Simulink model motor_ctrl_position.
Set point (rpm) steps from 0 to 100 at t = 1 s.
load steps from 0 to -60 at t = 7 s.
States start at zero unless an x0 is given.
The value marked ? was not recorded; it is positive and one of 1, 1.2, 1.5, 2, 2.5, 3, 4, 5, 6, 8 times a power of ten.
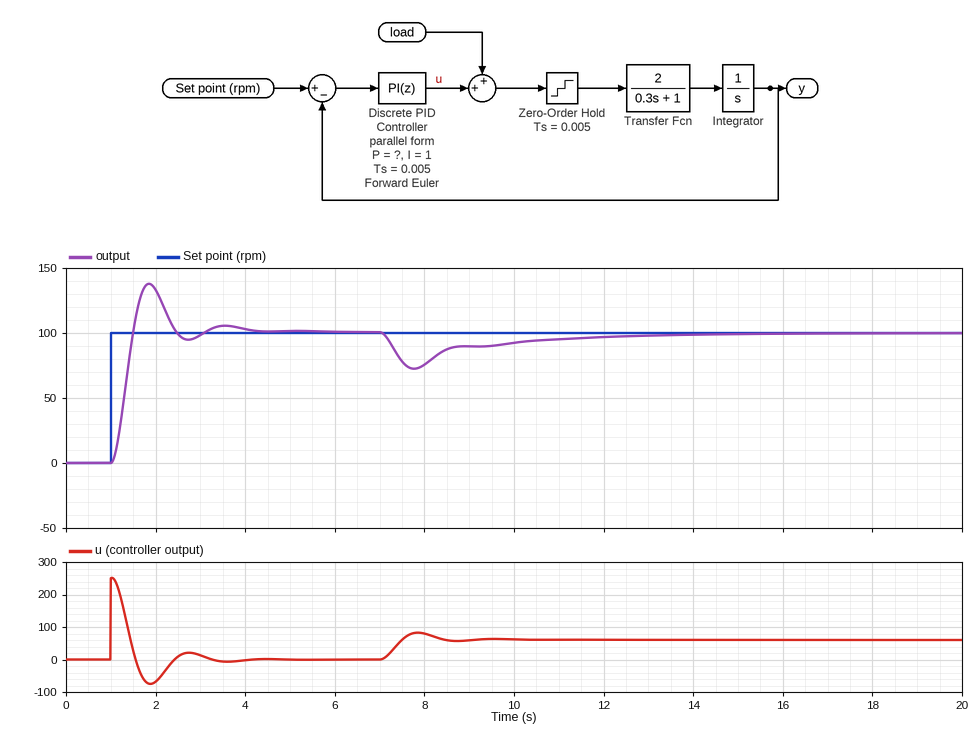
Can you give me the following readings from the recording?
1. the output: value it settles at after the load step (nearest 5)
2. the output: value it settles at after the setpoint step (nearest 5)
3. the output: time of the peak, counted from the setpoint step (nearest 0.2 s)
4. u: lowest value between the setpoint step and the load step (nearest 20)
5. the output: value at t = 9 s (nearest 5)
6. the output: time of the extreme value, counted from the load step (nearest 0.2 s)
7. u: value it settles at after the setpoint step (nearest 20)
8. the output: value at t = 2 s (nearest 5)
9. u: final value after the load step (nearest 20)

100
100
0.8 s
-80
90
0.8 s
0
135
60
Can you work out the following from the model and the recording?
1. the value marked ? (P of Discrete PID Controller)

2.5
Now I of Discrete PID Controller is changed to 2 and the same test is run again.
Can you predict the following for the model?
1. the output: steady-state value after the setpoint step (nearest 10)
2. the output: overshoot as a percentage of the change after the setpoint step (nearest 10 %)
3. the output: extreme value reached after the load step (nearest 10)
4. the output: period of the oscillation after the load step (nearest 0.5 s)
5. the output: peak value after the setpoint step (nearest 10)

100
50 %
70
1.5 s
150
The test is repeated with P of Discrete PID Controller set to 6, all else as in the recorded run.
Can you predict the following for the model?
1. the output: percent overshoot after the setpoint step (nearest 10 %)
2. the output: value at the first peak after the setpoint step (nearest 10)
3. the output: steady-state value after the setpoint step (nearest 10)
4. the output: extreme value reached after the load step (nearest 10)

50 %
150
100
90
